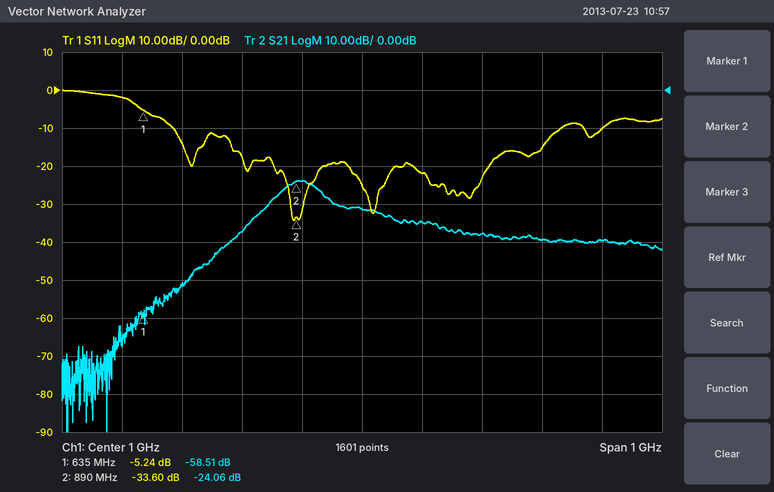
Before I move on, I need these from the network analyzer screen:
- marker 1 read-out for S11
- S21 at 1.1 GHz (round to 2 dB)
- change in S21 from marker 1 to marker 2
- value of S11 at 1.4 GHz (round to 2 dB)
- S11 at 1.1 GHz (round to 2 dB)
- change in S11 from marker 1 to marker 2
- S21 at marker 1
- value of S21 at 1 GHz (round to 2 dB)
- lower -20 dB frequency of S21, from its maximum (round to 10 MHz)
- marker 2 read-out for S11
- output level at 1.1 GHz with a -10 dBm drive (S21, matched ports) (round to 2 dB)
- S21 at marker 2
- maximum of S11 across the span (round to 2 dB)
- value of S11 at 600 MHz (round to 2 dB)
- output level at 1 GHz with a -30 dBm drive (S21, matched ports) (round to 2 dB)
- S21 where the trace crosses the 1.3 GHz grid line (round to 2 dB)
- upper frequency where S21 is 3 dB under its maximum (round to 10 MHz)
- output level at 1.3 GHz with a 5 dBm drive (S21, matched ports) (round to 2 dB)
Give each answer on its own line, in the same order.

-5.24 dB
-34 dB
34.45 dB
-10 dB
-22 dB
-28.36 dB
-58.51 dB
-32 dB
750 MHz
-33.60 dB
-44 dBm
-24.06 dB
0 dB
-2 dB
-62 dBm
-40 dB
930 MHz
-34 dBm
